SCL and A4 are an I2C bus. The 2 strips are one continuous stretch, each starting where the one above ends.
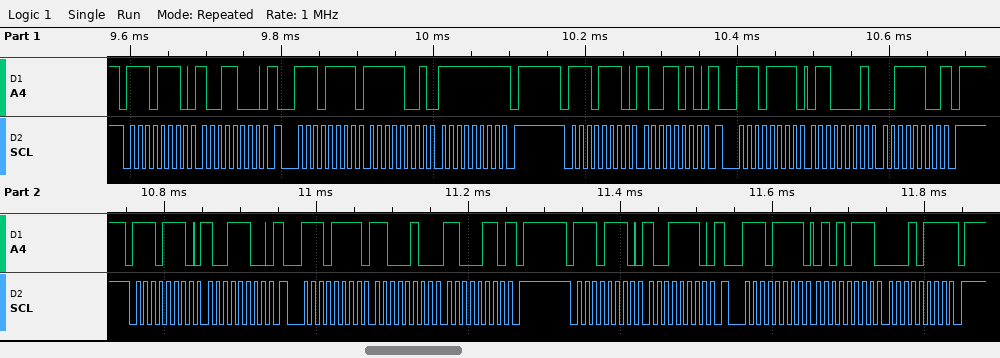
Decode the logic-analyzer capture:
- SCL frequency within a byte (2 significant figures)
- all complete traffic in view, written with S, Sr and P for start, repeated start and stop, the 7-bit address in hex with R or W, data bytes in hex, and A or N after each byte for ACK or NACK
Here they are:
100 kHz
S 77W A 98 A Sr 77R A F9 A FF N P S 77W A 9A A Sr 77R A 61 A 3C N P S 77W A 9C A Sr 77R A C4 A C6 N P S 77W A 9E A Sr 77R A 57 A 17 N P
